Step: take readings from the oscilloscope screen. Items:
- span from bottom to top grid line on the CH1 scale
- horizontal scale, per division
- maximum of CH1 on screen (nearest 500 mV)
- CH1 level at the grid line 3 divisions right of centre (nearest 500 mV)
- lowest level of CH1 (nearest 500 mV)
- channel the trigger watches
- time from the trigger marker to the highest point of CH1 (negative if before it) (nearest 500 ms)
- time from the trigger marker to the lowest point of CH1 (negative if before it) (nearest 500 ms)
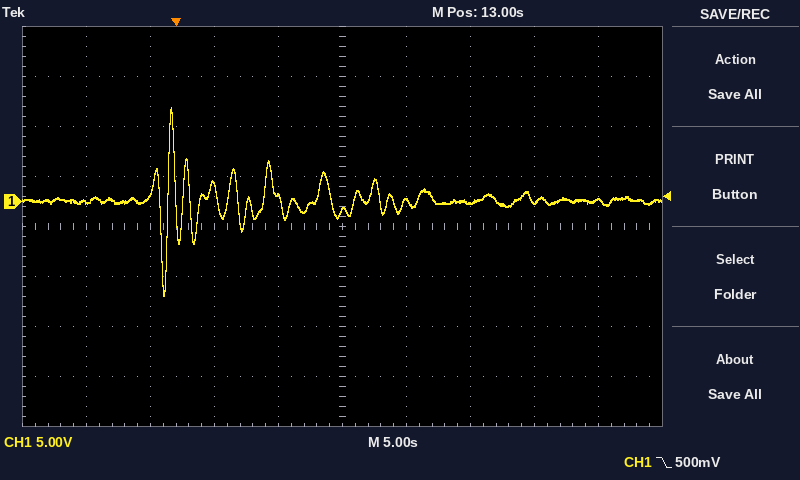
40 V
5 s
9.5 V
0.0 V
-9.5 V
CH1
-500 ms
-1.0 s
